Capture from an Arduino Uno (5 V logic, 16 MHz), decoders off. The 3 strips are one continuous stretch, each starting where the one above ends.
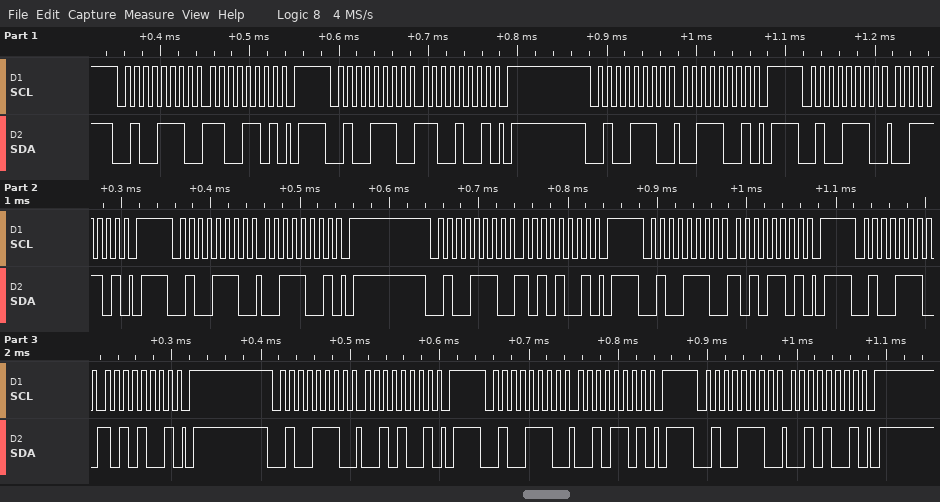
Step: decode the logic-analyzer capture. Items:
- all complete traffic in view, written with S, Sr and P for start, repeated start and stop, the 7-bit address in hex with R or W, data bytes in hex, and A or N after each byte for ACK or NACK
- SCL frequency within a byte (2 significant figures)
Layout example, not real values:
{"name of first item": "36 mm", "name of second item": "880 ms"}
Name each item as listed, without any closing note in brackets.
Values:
{"all complete traffic in view, written with S, Sr and P for start, repeated start and stop, the 7-bit address in hex with R or W, data bytes in hex, and A or N after each byte for ACK or NACK": "S 27W A CD A P S 27W A C9 A P S 27W A 39 A P S 27W A 3D A P S 27W A 39 A P S 27W A A9 A P S 27W A AD A P S 27W A A9 A P S 27W A 29 A P S 27W A 2D A P S 27W A 29 A P", "SCL frequency within a byte": "100 kHz"}
